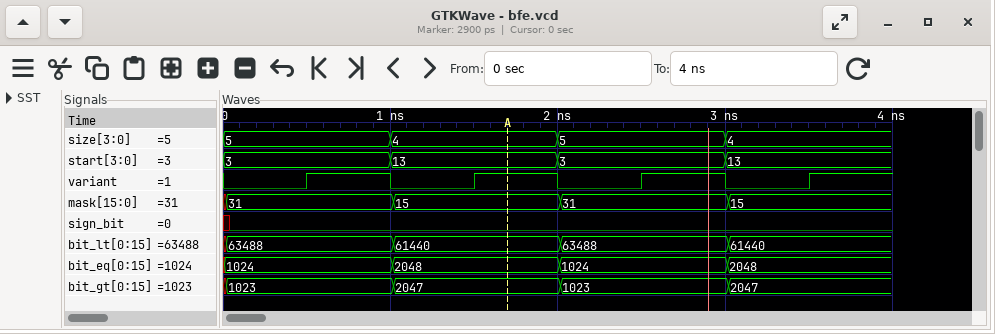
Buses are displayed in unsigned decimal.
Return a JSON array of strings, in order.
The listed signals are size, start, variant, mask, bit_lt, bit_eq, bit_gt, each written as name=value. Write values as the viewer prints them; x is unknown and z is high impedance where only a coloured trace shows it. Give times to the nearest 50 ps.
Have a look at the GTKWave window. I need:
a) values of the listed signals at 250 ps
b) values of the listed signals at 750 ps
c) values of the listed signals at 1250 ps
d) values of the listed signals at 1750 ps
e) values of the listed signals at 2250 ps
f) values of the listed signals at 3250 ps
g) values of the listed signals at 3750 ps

["size=5, start=3, variant=0, mask=31, bit_lt=63488, bit_eq=1024, bit_gt=1023", "size=5, start=3, variant=1, mask=31, bit_lt=63488, bit_eq=1024, bit_gt=1023", "size=4, start=13, variant=0, mask=15, bit_lt=61440, bit_eq=2048, bit_gt=2047", "size=4, start=13, variant=1, mask=15, bit_lt=61440, bit_eq=2048, bit_gt=2047", "size=5, start=3, variant=0, mask=31, bit_lt=63488, bit_eq=1024, bit_gt=1023", "size=4, start=13, variant=0, mask=15, bit_lt=61440, bit_eq=2048, bit_gt=2047", "size=4, start=13, variant=1, mask=15, bit_lt=61440, bit_eq=2048, bit_gt=2047"]
